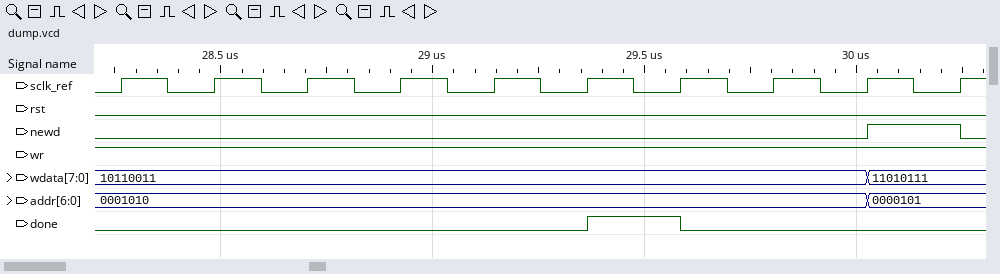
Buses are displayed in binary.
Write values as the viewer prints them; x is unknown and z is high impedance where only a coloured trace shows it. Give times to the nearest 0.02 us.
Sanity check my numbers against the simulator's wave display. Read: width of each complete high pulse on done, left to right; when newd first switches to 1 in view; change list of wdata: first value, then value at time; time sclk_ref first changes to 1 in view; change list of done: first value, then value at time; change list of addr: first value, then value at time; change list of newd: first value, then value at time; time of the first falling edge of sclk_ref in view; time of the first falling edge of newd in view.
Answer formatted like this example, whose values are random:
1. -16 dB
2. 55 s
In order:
1. 0.22 us
2. 30.02 us
3. 10110011, 11010111 at 30.02 us
4. 28.26 us
5. 0, 1 at 29.36 us, 0 at 29.58 us
6. 0001010, 0000101 at 30.02 us
7. 0, 1 at 30.02 us, 0 at 30.24 us
8. 28.38 us
9. 30.24 us
